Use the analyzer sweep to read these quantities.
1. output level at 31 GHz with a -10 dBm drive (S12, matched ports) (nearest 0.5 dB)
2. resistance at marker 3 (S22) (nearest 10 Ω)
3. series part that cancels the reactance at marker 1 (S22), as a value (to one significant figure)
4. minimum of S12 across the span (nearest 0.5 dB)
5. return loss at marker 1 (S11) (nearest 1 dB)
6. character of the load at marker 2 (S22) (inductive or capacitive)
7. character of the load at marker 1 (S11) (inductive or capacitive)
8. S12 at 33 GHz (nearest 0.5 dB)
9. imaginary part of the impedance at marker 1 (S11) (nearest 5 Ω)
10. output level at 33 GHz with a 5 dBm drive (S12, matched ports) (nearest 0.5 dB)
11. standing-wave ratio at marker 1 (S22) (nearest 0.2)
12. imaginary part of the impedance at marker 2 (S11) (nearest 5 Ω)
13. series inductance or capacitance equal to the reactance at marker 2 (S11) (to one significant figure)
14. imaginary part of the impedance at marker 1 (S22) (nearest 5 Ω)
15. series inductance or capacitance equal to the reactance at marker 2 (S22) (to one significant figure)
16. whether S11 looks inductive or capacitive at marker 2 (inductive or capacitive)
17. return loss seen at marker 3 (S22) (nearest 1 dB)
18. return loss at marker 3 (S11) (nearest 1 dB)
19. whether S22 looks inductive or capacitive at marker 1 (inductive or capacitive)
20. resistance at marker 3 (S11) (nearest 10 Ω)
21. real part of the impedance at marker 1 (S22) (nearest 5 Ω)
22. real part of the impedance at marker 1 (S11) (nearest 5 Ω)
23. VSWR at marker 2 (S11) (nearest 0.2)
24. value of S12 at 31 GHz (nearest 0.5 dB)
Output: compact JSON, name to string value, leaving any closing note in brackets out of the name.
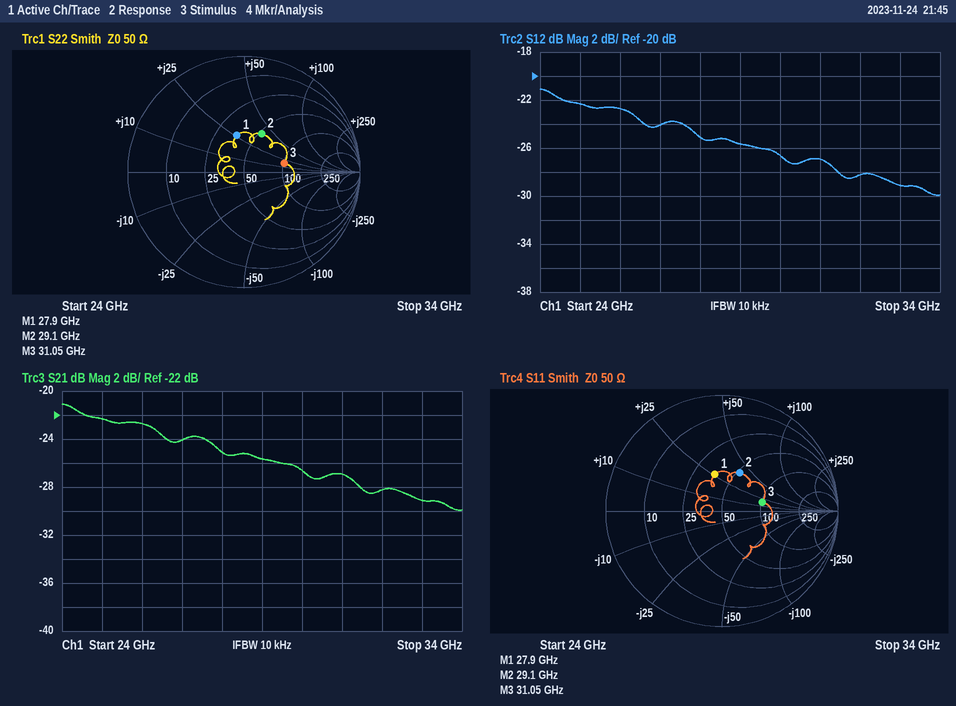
{"output level at 31 GHz with a -10 dBm drive (S12, matched ports)": "-37.0 dBm", "resistance at marker 3 (S22)": "100 Ω", "series part that cancels the reactance at marker 1 (S22), as a value": "200 fF", "minimum of S12 across the span": "-30.0 dB", "return loss at marker 1 (S11)": "10 dB", "character of the load at marker 2 (S22)": "inductive", "character of the load at marker 1 (S11)": "inductive", "S12 at 33 GHz": "-29.0 dB", "imaginary part of the impedance at marker 1 (S11)": "+25 Ω", "output level at 33 GHz with a 5 dBm drive (S12, matched ports)": "-24.0 dBm", "standing-wave ratio at marker 1 (S22)": "2.0", "imaginary part of the impedance at marker 2 (S11)": "+40 Ω", "series inductance or capacitance equal to the reactance at marker 2 (S11)": "200 pH", "imaginary part of the impedance at marker 1 (S22)": "+25 Ω", "series inductance or capacitance equal to the reactance at marker 2 (S22)": "200 pH", "whether S11 looks inductive or capacitive at marker 2": "inductive", "return loss seen at marker 3 (S22)": "9 dB", "return loss at marker 3 (S11)": "9 dB", "whether S22 looks inductive or capacitive at marker 1": "inductive", "resistance at marker 3 (S11)": "100 Ω", "real part of the impedance at marker 1 (S22)": "35 Ω", "real part of the impedance at marker 1 (S11)": "35 Ω", "VSWR at marker 2 (S11)": "2.2", "value of S12 at 31 GHz": "-27.0 dB"}
